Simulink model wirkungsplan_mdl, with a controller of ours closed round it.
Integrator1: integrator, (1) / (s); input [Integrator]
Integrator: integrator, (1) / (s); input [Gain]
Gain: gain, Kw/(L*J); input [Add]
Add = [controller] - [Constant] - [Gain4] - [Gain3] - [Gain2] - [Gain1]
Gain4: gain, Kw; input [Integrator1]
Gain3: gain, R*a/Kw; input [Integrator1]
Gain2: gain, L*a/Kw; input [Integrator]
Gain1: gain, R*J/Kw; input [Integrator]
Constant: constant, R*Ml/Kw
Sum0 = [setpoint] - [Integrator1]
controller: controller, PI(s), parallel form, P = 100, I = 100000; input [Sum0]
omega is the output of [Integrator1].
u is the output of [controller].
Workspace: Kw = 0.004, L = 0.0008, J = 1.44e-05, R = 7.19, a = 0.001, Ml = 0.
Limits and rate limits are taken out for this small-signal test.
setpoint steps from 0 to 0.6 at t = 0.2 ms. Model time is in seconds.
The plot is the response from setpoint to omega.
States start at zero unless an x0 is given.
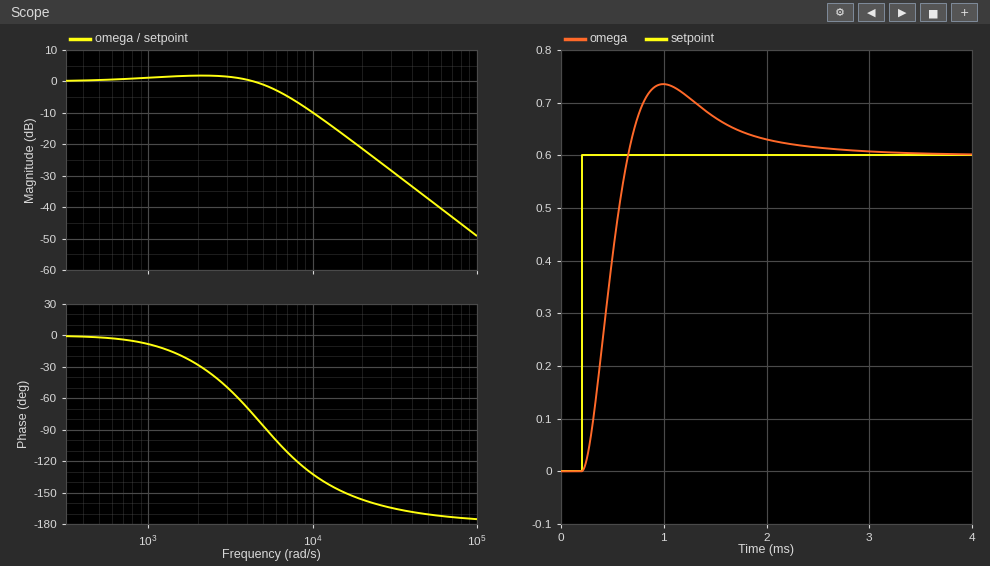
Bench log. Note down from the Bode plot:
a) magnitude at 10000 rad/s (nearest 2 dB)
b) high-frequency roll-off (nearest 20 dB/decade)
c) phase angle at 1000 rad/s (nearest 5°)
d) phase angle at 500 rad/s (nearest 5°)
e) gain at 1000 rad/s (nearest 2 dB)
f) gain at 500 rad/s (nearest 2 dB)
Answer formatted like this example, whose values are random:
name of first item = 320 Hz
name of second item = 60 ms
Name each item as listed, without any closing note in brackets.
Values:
magnitude at 10000 rad/s = -10 dB
high-frequency roll-off = -40 dB/decade
phase angle at 1000 rad/s = -10°
phase angle at 500 rad/s = 0°
gain at 1000 rad/s = 2 dB
gain at 500 rad/s = 0 dB
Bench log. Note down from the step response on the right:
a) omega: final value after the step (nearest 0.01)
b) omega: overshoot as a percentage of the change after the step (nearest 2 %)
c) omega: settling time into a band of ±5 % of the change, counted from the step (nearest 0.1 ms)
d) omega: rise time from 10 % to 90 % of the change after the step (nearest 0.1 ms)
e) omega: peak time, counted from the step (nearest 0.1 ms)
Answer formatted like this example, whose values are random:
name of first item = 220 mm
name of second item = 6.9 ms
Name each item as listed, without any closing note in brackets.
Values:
omega: final value after the step = 0.60
omega: overshoot as a percentage of the change after the step = 22 %
omega: settling time into a band of ±5 % of the change, counted from the step = 1.8 ms
omega: rise time from 10 % to 90 % of the change after the step = 0.3 ms
omega: peak time, counted from the step = 0.8 ms
